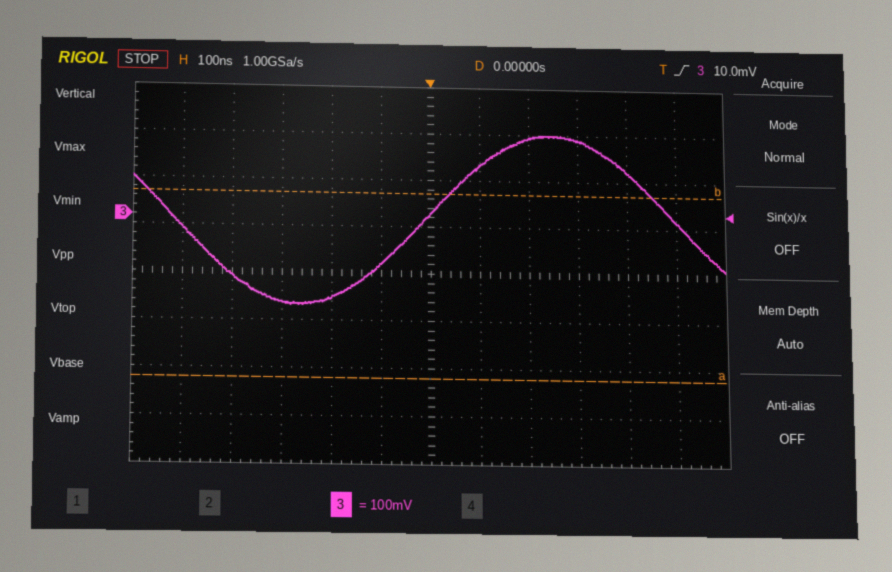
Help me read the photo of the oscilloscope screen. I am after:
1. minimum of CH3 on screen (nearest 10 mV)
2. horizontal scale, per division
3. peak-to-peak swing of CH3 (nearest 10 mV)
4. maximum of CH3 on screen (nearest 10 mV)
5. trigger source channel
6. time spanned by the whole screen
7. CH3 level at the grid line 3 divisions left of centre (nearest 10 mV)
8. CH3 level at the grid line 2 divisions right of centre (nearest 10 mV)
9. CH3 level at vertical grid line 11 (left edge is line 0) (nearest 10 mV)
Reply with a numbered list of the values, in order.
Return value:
1. -190 mV
2. 100 ns
3. 370 mV
4. 180 mV
5. CH3
6. 1.2 µs
7. -180 mV
8. 170 mV
9. 0 mV
